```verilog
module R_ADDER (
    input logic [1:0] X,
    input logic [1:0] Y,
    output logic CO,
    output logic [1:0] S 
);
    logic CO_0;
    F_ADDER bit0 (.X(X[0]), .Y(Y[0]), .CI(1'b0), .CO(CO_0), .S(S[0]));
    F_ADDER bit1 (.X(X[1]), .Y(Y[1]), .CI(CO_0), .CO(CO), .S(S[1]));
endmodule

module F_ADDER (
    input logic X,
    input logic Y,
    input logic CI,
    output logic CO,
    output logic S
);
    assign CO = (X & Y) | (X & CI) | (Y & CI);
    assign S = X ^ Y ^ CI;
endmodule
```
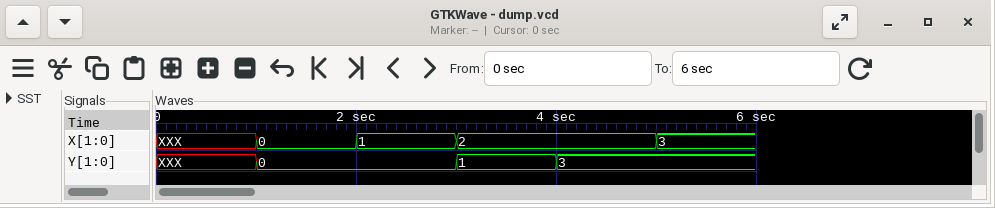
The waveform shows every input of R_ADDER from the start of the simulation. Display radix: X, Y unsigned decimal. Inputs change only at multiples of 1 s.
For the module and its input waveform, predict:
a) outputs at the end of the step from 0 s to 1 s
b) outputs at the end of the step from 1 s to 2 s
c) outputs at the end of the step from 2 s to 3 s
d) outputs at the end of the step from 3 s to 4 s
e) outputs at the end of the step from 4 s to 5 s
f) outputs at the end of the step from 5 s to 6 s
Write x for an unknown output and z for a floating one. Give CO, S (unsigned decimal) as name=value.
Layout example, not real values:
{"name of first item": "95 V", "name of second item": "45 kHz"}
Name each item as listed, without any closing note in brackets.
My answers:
{"outputs at the end of the step from 0 s to 1 s": "CO=x, S=x", "outputs at the end of the step from 1 s to 2 s": "CO=0, S=0", "outputs at the end of the step from 2 s to 3 s": "CO=0, S=1", "outputs at the end of the step from 3 s to 4 s": "CO=0, S=3", "outputs at the end of the step from 4 s to 5 s": "CO=1, S=1", "outputs at the end of the step from 5 s to 6 s": "CO=1, S=2"}
